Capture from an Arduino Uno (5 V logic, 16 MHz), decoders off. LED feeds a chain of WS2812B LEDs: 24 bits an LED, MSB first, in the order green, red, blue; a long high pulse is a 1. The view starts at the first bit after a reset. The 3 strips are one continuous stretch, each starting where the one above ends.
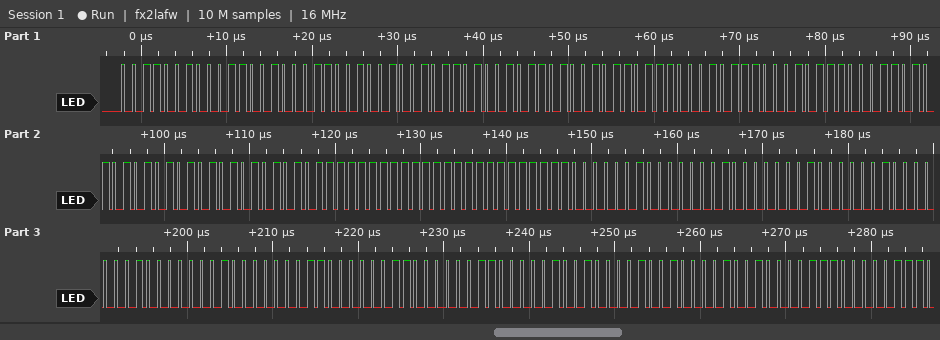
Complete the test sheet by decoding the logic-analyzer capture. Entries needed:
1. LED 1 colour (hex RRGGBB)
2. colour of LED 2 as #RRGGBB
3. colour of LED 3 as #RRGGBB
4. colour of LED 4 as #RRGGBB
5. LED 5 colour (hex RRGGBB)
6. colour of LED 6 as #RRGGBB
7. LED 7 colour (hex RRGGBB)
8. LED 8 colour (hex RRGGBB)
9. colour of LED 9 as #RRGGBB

#323232
#4B4B4B
#717171
#AAAAAA
#FFFFFF
#020202
#040404
#060606
#090909
